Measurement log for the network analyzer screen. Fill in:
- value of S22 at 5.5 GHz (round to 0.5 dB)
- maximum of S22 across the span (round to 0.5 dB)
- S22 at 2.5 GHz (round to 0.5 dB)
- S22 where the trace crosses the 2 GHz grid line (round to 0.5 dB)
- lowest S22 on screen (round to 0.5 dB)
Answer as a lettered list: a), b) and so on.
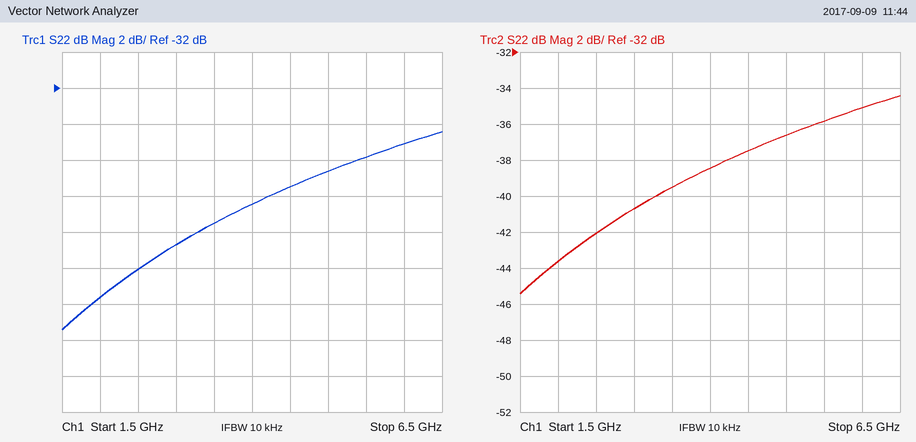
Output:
a) -36.0 dB
b) -34.5 dB
c) -42.0 dB
d) -43.5 dB
e) -45.5 dB
